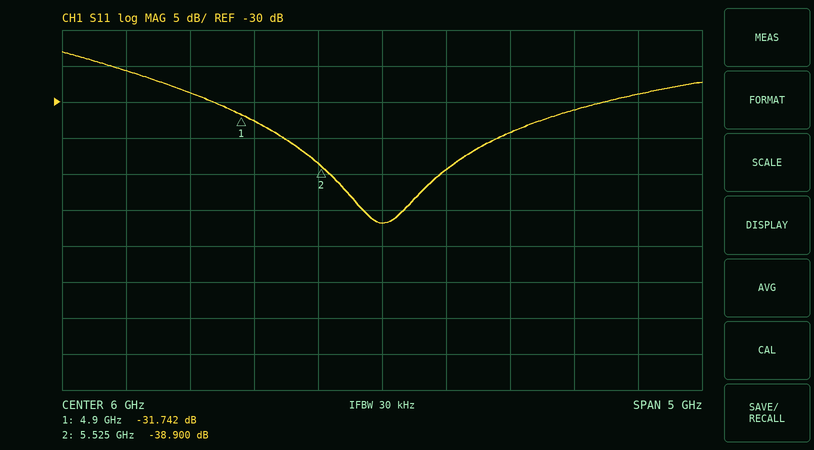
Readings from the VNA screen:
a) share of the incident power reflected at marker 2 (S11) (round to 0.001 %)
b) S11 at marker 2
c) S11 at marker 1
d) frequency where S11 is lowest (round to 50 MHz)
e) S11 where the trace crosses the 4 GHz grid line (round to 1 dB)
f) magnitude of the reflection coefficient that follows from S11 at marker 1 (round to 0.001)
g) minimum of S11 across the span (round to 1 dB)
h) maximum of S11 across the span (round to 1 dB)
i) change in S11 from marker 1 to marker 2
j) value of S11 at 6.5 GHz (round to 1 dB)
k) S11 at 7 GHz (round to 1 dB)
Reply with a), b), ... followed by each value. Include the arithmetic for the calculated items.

a) 10^(-38.9/10) ≈ 0.013 %
b) -38.900 dB
c) -31.742 dB
d) 6.00 GHz
e) -26 dB
f) 10^(-31.742/20) ≈ 0.026
g) -47 dB
h) -23 dB
i) -38.9 − (-31.742) = -7.158 dB
j) -39 dB
k) -34 dB
